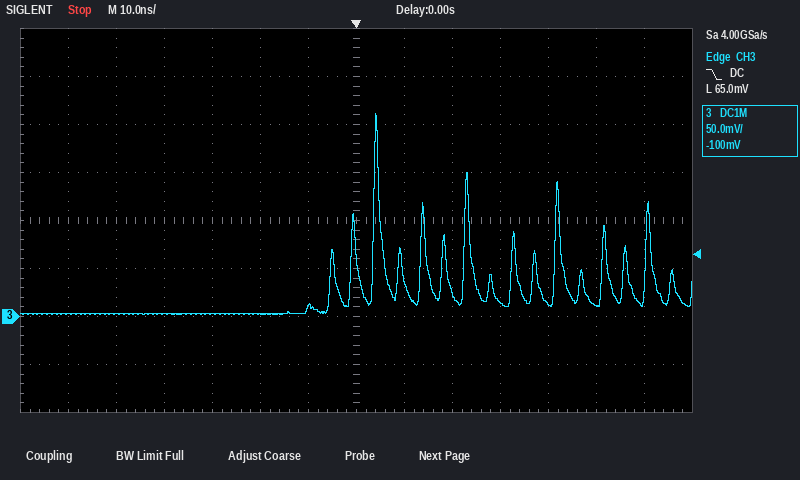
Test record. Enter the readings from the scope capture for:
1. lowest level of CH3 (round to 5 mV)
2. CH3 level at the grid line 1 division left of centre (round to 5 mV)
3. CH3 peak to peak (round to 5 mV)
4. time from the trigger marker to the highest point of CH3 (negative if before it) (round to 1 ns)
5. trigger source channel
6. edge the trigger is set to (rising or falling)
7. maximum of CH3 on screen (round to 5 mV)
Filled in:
0 mV
10 mV
210 mV
+4 ns
CH3
falling
210 mV
